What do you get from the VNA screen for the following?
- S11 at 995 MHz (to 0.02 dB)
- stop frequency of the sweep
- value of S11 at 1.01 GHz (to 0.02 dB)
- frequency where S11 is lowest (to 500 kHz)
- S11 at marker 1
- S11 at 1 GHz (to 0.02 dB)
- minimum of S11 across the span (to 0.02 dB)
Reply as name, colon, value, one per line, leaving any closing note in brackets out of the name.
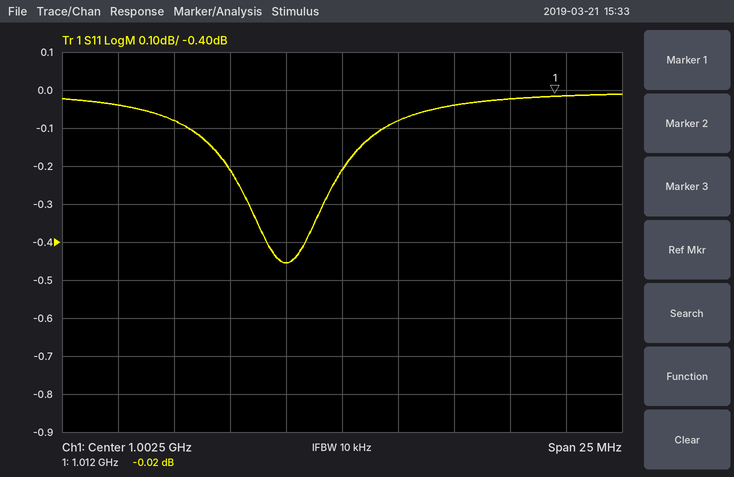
S11 at 995 MHz: -0.08 dB
stop frequency of the sweep: 1.015 GHz
value of S11 at 1.01 GHz: -0.02 dB
frequency where S11 is lowest: 1.0000 GHz
S11 at marker 1: -0.02 dB
S11 at 1 GHz: -0.46 dB
minimum of S11 across the span: -0.46 dB
